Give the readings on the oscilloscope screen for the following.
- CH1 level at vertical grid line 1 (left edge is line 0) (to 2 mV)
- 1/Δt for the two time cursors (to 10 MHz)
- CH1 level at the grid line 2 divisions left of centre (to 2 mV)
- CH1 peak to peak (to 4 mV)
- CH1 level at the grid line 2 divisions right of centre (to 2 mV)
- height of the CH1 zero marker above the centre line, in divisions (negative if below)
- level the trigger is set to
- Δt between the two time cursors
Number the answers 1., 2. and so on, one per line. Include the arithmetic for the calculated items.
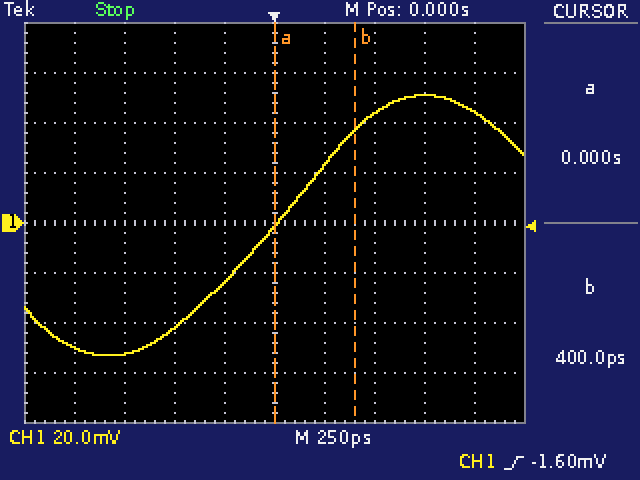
1. -50 mV
2. 1 / 400 ps ≈ 2.50 GHz
3. -42 mV
4. 104 mV
5. 44 mV
6. 0.0 div
7. -1.60 mV
8. 400 ps − (0 s) = 400 ps
